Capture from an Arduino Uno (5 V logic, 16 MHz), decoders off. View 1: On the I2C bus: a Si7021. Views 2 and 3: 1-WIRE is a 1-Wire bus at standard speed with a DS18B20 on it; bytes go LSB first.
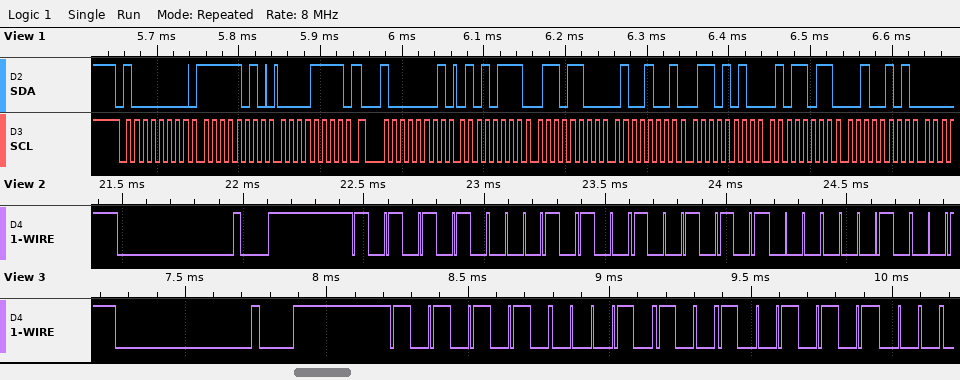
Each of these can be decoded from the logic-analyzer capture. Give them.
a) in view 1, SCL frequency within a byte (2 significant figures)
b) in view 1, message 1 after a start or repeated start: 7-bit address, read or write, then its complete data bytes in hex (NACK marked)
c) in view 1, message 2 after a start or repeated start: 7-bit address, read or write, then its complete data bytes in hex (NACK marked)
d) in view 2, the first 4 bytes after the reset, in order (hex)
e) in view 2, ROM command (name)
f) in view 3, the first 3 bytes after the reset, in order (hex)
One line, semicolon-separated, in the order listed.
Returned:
100 kHz; 0x40 write: FA 0F; 0x40 read: 57 6C 49 6A 5B 25; 55 28 A9 40; Match ROM; 55 28 A9
